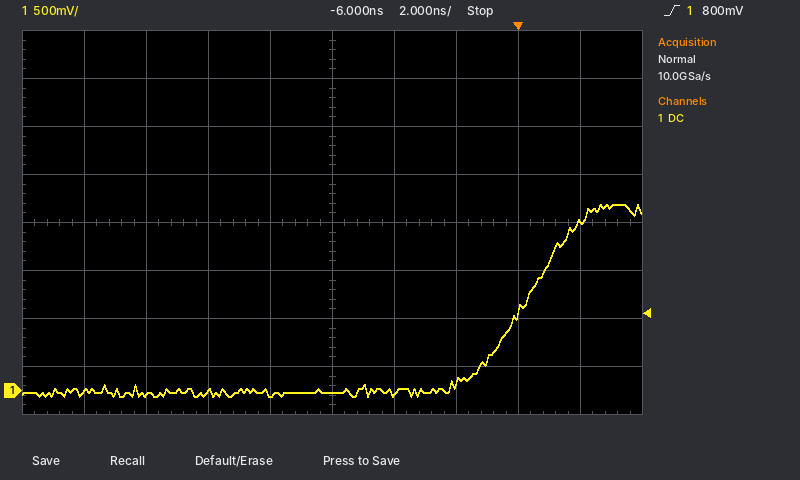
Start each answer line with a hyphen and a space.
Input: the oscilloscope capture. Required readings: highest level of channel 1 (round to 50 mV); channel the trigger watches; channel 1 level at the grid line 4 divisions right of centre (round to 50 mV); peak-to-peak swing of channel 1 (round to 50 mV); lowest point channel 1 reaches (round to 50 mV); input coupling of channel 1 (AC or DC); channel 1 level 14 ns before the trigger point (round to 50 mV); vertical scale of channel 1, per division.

- 1.95 V
- channel 1
- 1.75 V
- 2.00 V
- -50 mV
- DC
- 0 mV
- 500 mV
